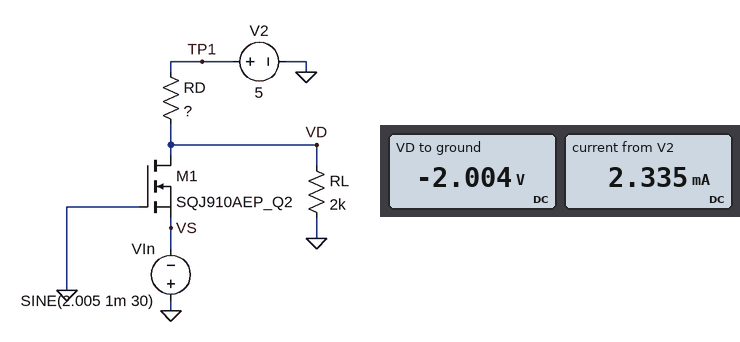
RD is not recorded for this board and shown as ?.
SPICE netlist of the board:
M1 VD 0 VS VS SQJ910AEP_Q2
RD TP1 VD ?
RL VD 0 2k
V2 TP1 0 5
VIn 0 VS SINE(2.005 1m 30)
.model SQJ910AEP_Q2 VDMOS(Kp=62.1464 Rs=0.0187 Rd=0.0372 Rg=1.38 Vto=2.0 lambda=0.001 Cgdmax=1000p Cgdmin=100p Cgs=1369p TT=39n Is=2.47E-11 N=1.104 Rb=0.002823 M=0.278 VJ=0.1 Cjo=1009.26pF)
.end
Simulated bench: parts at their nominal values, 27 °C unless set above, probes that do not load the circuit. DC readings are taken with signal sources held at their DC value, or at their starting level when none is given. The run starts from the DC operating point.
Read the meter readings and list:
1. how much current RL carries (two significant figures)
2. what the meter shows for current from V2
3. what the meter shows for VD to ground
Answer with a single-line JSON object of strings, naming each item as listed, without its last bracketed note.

{"how much current RL carries": "1.0 mA", "what the meter shows for current from V2": "2.335 mA", "what the meter shows for VD to ground": "-2.004 V"}
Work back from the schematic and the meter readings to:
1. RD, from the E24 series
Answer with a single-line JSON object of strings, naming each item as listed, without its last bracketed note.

{"RD, from the E24 series": "3 kΩ"}
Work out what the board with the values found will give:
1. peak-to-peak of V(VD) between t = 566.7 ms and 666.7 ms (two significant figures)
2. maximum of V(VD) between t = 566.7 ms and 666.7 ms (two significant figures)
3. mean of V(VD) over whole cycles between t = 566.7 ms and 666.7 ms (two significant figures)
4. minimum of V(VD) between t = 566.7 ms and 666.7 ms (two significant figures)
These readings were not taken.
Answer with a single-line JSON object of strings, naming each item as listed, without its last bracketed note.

{"peak-to-peak of V(VD) between t = 566.7 ms and 666.7 ms": "2.0 mV", "maximum of V(VD) between t = 566.7 ms and 666.7 ms": "-2.0 V", "mean of V(VD) over whole cycles between t = 566.7 ms and 666.7 ms": "-2.0 V", "minimum of V(VD) between t = 566.7 ms and 666.7 ms": "-2.0 V"}
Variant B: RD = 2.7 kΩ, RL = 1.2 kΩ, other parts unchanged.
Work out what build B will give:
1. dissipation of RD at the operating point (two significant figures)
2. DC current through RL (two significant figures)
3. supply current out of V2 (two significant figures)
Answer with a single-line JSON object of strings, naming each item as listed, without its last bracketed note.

{"dissipation of RD at the operating point": "18 mW", "DC current through RL": "1.7 mA", "supply current out of V2": "2.6 mA"}
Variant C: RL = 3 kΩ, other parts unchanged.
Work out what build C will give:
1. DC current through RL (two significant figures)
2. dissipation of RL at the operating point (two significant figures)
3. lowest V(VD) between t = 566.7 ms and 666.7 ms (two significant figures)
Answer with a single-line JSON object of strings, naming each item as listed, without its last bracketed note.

{"DC current through RL": "670 µA", "dissipation of RL at the operating point": "1.3 mW", "lowest V(VD) between t = 566.7 ms and 666.7 ms": "-2.0 V"}
